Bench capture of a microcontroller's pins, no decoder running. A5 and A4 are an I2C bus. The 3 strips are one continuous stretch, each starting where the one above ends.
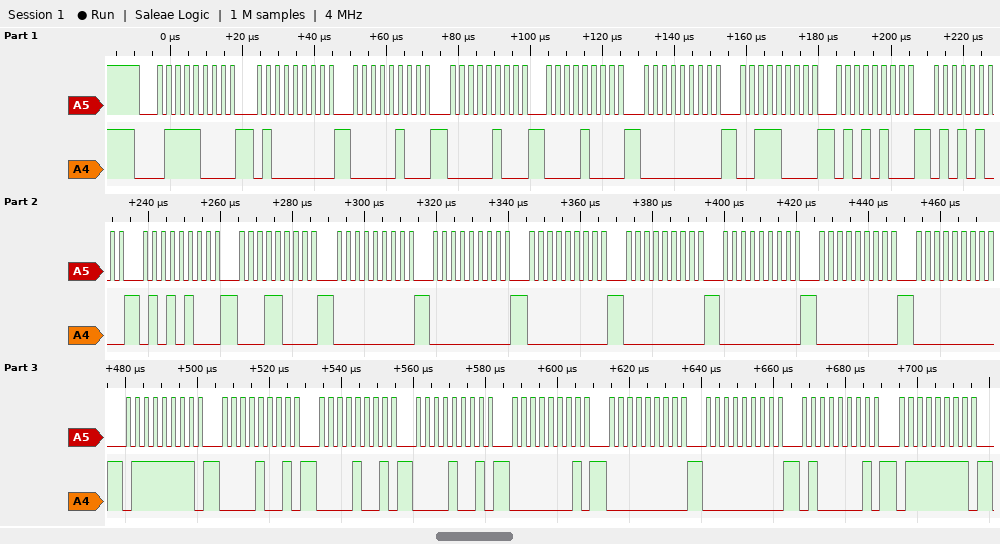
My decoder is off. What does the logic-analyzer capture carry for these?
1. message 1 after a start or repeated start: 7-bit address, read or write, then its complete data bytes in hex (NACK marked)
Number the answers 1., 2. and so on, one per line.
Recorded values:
1. 0x3C write: 40 04 04 08 00 38 54 54 54 18 00 00 00 00 00 00 00 7F 09 09 09 01 00 00 41 7F
